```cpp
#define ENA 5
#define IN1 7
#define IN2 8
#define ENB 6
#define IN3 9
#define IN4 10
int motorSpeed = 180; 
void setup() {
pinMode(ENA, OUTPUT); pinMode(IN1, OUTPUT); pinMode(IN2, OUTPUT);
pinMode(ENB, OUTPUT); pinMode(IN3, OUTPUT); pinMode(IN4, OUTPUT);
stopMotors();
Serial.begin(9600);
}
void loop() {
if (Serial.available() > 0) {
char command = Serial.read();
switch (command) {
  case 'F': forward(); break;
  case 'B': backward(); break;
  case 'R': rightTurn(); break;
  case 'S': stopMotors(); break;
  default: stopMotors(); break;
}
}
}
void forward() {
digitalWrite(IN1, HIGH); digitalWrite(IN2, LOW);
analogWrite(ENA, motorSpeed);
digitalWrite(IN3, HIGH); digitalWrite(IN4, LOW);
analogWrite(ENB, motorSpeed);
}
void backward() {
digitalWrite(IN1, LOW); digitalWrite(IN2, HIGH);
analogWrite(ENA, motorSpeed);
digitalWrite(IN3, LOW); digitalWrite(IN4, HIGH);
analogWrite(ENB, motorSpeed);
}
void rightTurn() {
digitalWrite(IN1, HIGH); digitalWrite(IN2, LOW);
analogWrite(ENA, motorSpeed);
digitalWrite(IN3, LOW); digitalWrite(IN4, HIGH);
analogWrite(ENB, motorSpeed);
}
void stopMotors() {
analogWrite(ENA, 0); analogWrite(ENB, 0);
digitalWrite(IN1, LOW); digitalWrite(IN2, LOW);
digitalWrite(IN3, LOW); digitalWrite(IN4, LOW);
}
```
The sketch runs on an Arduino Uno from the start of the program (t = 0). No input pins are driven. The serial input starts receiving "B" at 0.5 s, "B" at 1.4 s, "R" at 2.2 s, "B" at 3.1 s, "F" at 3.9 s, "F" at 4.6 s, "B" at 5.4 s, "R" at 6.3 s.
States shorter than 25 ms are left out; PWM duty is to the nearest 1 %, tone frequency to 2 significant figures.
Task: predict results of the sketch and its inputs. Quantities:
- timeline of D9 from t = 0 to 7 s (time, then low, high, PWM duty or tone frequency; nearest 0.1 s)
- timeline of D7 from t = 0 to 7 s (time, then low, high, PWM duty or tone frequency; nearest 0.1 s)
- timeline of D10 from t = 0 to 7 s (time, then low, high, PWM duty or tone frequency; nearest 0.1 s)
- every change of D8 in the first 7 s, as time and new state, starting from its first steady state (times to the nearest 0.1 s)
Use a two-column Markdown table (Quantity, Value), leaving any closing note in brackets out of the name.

| Quantity | Value |
|---|---|
| timeline of D9 from t = 0 to 7 s | 0 s low; 3.9 s high; 5.4 s low |
| timeline of D7 from t = 0 to 7 s | 0 s low; 2.2 s high; 3.1 s low; 3.9 s high; 5.4 s low; 6.3 s high |
| timeline of D10 from t = 0 to 7 s | 0 s low; 0.5 s high; 3.9 s low; 5.4 s high |
| every change of D8 in the first 7 s, as time and new state, starting from its first steady state | 0 s low; 0.5 s high; 2.2 s low; 3.1 s high; 3.9 s low; 5.4 s high; 6.3 s low |
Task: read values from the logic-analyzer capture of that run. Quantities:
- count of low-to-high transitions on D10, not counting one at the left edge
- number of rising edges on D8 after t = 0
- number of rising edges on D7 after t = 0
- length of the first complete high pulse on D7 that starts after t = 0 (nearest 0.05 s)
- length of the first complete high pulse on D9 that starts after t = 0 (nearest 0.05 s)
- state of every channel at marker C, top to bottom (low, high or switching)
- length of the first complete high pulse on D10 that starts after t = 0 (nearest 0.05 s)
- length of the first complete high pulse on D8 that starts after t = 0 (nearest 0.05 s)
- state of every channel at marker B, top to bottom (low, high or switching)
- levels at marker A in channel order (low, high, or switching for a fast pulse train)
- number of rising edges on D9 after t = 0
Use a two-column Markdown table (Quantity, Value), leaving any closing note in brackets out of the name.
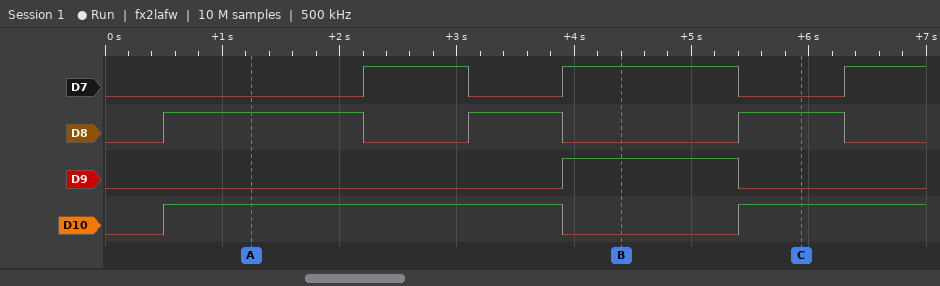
| Quantity | Value |
|---|---|
| count of low-to-high transitions on D10, not counting one at the left edge | 2 |
| number of rising edges on D8 after t = 0 | 3 |
| number of rising edges on D7 after t = 0 | 3 |
| length of the first complete high pulse on D7 that starts after t = 0 | 0.90 s |
| length of the first complete high pulse on D9 that starts after t = 0 | 1.50 s |
| state of every channel at marker C, top to bottom | D7 low, D8 high, D9 low, D10 high |
| length of the first complete high pulse on D10 that starts after t = 0 | 3.40 s |
| length of the first complete high pulse on D8 that starts after t = 0 | 1.70 s |
| state of every channel at marker B, top to bottom | D7 high, D8 low, D9 high, D10 low |
| levels at marker A in channel order | D7 low, D8 high, D9 low, D10 high |
| number of rising edges on D9 after t = 0 | 1 |
